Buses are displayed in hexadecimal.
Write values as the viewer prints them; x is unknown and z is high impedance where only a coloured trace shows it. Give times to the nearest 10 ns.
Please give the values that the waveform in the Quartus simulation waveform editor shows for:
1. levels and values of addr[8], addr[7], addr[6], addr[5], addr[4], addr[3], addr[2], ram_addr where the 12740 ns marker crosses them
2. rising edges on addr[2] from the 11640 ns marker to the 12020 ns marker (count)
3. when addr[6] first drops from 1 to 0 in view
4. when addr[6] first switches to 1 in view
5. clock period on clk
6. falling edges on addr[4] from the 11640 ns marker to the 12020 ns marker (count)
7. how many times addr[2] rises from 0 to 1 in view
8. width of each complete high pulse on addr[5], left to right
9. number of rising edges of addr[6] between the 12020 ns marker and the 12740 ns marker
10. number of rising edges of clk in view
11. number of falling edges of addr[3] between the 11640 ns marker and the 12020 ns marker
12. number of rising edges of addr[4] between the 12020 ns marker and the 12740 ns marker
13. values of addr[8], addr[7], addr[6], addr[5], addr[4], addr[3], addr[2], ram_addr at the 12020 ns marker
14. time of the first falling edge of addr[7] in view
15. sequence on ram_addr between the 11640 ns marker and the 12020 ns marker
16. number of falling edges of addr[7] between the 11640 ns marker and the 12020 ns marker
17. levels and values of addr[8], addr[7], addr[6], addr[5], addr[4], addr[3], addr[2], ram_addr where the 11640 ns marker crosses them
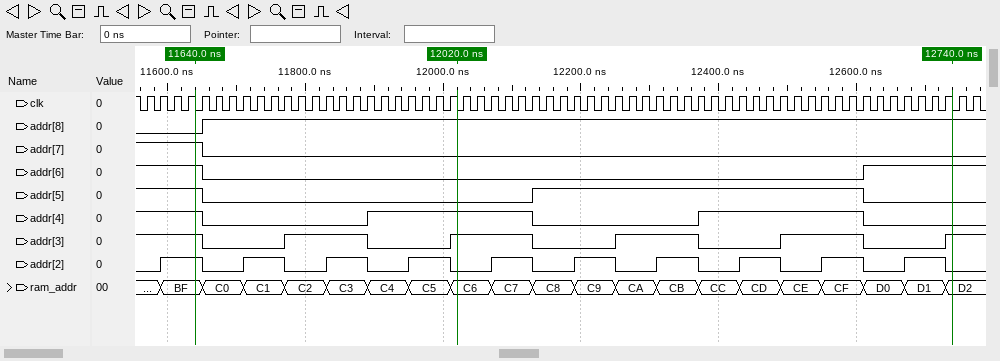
addr[8]=1, addr[7]=0, addr[6]=1, addr[5]=0, addr[4]=0, addr[3]=1, addr[2]=0, ram_addr=D2
3
11650 ns
12610 ns
20 ns
1
10
480 ns
1
61
2
1
addr[8]=1, addr[7]=0, addr[6]=0, addr[5]=0, addr[4]=1, addr[3]=1, addr[2]=0, ram_addr=C6
11650 ns
BF, C0, C1, C2, C3, C4, C5, C6
1
addr[8]=0, addr[7]=1, addr[6]=1, addr[5]=1, addr[4]=1, addr[3]=1, addr[2]=1, ram_addr=BF
